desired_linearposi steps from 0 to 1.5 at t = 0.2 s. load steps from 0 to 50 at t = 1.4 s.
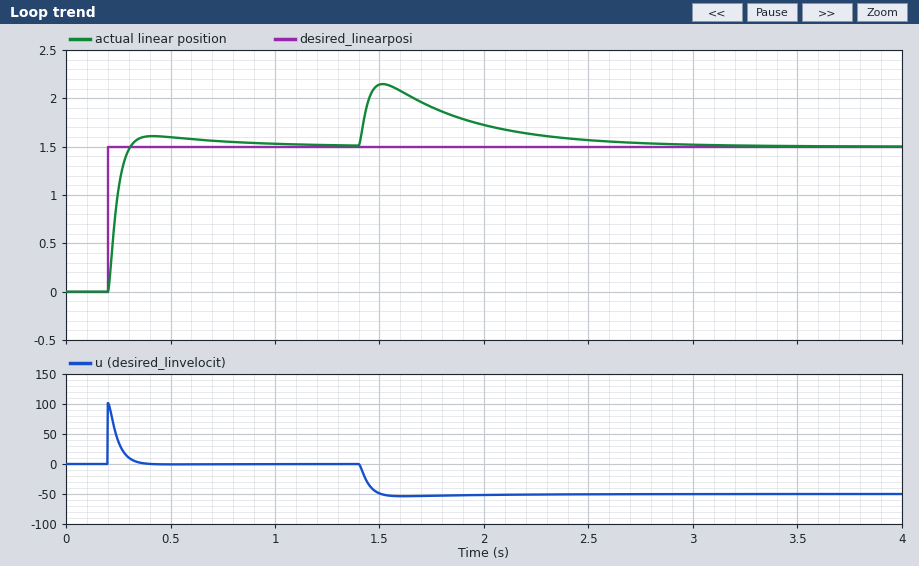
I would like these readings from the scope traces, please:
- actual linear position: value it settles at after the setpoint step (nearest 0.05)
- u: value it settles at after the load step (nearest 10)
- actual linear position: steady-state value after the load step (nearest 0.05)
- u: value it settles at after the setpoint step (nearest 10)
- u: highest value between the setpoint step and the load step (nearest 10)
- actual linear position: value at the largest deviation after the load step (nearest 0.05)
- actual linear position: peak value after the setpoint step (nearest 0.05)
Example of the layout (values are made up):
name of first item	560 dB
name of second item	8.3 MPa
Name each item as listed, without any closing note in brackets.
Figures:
actual linear position: value it settles at after the setpoint step	1.50
u: value it settles at after the load step	-50
actual linear position: steady-state value after the load step	1.50
u: value it settles at after the setpoint step	0
u: highest value between the setpoint step and the load step	100
actual linear position: value at the largest deviation after the load step	2.15
actual linear position: peak value after the setpoint step	1.60
